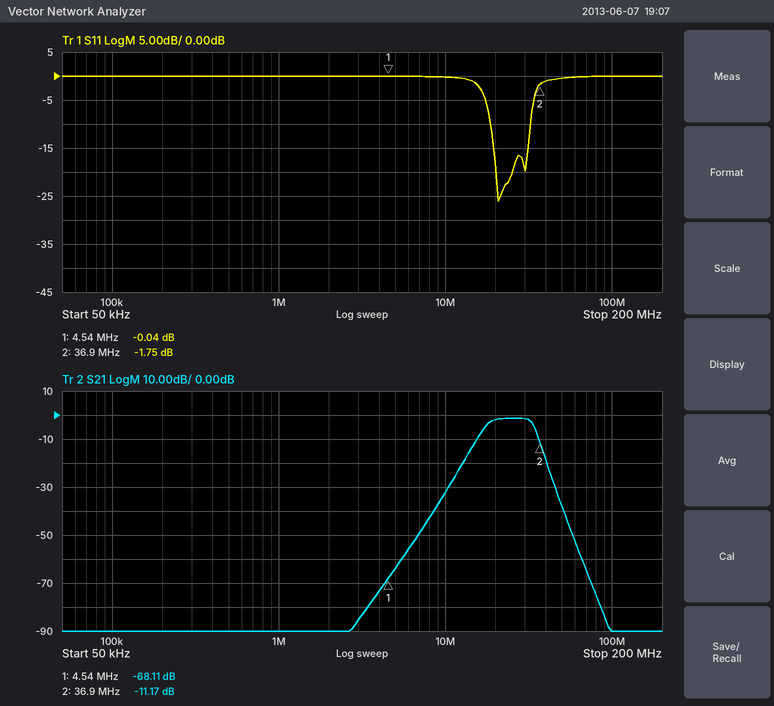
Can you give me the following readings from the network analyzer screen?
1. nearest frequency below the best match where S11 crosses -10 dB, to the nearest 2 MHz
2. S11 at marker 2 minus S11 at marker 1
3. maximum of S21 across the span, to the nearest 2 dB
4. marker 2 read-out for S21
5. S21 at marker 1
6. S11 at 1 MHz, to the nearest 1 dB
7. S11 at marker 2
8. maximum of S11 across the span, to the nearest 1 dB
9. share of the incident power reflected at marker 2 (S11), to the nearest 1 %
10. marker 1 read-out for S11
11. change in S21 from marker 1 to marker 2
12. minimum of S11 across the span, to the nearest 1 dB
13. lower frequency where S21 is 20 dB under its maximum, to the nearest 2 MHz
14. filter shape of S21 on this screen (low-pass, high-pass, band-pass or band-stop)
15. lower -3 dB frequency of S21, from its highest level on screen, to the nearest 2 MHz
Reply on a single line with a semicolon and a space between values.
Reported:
18 MHz; -1.71 dB; -2 dB; -11.17 dB; -68.11 dB; 0 dB; -1.75 dB; 0 dB; 67 %; -0.04 dB; 56.94 dB; -26 dB; 12 MHz; band-pass; 18 MHz
